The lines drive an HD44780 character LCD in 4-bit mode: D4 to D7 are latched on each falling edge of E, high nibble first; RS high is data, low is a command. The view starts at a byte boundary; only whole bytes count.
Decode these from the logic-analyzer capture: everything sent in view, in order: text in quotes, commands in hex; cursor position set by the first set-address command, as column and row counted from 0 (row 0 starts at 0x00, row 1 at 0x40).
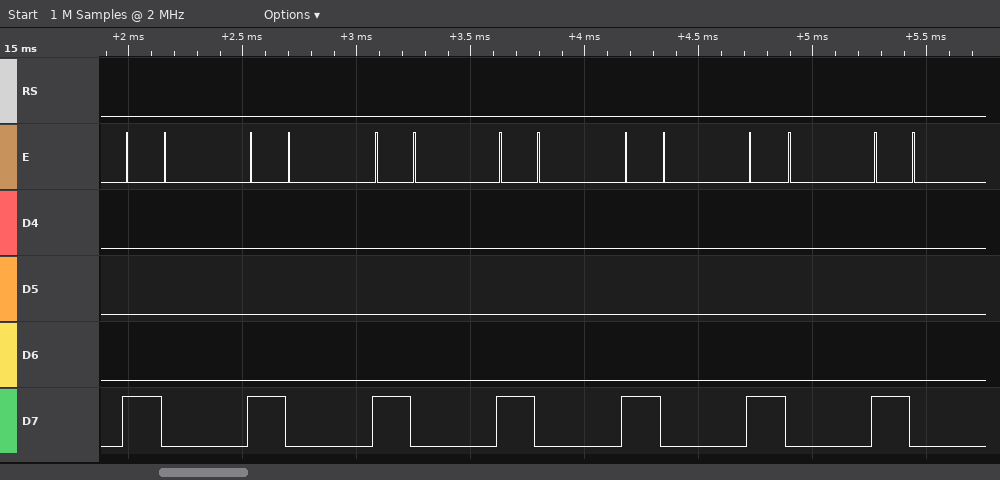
0x80 0x80 0x80 0x80 0x80 0x80 0x80
column 0, row 0
